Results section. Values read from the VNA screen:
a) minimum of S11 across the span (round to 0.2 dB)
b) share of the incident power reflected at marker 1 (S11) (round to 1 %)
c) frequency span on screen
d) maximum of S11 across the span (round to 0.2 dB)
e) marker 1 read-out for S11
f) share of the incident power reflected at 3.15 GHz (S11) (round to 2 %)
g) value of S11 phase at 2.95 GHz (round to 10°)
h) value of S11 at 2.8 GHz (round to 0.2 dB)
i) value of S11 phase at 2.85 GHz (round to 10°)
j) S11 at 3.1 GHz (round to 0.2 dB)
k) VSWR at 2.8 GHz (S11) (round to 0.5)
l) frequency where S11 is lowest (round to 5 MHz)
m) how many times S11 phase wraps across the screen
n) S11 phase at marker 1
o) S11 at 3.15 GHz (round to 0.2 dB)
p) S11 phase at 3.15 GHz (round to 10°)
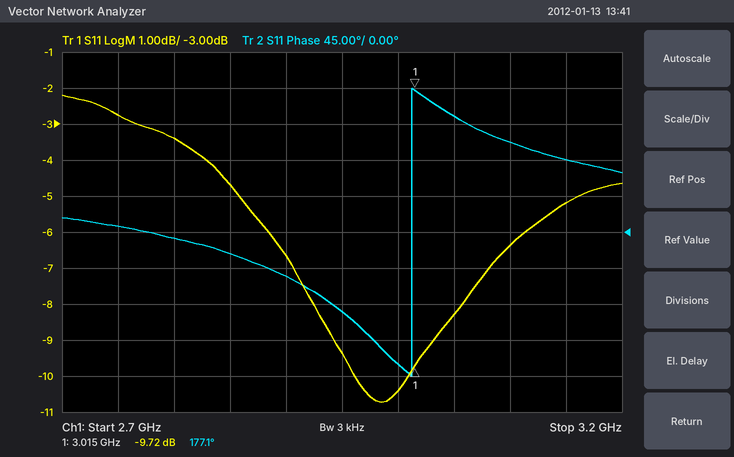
-10.8 dB
11 %
500 MHz
-2.2 dB
-9.72 dB
30 %
-100°
-3.4 dB
-30°
-6.4 dB
5.0
2.985 GHz
1
177.1°
-5.2 dB
90°
